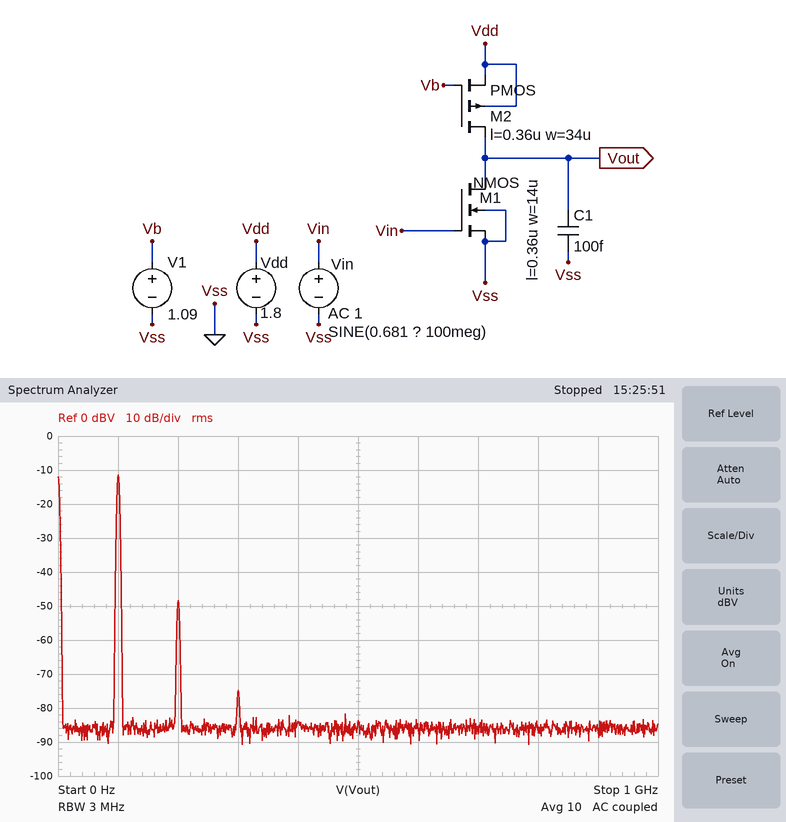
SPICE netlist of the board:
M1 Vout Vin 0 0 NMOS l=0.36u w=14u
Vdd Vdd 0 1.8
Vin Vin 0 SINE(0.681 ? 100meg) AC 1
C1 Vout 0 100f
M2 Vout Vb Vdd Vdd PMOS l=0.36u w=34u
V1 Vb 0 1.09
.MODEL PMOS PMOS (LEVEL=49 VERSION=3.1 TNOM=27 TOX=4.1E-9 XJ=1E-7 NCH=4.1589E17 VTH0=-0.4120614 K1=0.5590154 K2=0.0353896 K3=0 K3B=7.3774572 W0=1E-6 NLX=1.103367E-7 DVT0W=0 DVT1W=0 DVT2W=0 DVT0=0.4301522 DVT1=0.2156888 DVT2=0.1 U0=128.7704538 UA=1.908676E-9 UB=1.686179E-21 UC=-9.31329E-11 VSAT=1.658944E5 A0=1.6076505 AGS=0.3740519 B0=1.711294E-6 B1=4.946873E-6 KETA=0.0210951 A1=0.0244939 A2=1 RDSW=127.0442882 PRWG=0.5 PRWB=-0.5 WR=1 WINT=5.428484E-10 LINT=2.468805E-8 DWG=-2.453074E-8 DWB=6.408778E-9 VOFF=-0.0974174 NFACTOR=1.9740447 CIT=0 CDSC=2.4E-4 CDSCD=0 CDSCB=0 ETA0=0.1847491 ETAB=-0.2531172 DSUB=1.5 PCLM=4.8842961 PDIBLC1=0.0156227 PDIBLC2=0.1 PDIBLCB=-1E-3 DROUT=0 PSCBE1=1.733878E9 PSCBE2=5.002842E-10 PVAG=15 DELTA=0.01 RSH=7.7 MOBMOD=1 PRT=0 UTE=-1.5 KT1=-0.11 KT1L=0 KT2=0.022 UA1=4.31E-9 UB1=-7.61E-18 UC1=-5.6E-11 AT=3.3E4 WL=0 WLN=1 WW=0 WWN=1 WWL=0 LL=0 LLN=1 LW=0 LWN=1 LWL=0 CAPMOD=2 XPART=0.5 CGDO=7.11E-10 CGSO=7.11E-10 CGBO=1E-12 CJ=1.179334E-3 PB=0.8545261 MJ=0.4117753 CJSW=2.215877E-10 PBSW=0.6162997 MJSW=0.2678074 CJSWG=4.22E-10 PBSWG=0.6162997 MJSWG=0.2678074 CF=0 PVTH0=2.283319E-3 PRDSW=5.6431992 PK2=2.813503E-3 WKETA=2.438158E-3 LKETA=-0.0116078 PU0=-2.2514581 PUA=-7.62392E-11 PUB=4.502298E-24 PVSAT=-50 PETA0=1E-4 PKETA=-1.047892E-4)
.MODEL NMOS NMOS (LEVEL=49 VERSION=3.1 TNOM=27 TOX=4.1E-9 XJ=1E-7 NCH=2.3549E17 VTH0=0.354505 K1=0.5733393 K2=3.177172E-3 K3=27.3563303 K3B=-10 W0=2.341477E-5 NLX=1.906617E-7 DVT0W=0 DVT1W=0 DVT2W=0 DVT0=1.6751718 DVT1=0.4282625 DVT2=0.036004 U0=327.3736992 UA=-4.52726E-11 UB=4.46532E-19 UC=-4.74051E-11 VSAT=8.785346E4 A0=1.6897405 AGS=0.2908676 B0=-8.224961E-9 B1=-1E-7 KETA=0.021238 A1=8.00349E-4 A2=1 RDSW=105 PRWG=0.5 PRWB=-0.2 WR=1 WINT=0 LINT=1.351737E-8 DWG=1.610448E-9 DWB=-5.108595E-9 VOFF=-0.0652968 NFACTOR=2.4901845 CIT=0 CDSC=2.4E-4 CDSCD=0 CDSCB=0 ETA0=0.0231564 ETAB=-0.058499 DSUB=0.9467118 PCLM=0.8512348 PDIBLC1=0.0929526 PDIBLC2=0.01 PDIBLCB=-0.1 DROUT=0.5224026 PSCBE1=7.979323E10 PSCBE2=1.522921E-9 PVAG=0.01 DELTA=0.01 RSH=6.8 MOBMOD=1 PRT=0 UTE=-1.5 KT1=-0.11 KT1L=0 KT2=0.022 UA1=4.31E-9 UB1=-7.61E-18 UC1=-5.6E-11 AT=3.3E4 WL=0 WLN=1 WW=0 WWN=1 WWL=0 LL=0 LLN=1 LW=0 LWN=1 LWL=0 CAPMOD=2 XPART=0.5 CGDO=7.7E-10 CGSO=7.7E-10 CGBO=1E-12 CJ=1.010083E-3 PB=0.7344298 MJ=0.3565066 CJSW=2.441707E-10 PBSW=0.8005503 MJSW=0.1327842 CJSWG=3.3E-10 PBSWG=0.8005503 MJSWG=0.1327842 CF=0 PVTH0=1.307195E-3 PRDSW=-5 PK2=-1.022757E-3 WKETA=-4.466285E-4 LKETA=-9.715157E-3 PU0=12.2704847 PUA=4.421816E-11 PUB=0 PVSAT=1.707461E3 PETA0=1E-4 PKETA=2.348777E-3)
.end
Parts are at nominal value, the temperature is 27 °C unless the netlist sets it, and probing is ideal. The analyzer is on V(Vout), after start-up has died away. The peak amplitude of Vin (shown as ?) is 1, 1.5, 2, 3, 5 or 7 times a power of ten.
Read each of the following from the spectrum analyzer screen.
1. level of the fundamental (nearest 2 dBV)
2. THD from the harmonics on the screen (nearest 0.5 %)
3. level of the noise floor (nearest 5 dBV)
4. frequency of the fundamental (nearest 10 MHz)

-12 dBV
1.5 %
-85 dBV
100 MHz
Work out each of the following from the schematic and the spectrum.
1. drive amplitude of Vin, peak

20 mV
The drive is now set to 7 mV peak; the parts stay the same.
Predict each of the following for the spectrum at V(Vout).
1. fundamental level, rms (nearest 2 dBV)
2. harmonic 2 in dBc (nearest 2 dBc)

-20 dBV
-46 dBc
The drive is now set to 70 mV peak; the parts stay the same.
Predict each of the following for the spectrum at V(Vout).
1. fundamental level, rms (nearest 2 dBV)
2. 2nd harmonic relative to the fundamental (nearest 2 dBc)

-4 dBV
-26 dBc
